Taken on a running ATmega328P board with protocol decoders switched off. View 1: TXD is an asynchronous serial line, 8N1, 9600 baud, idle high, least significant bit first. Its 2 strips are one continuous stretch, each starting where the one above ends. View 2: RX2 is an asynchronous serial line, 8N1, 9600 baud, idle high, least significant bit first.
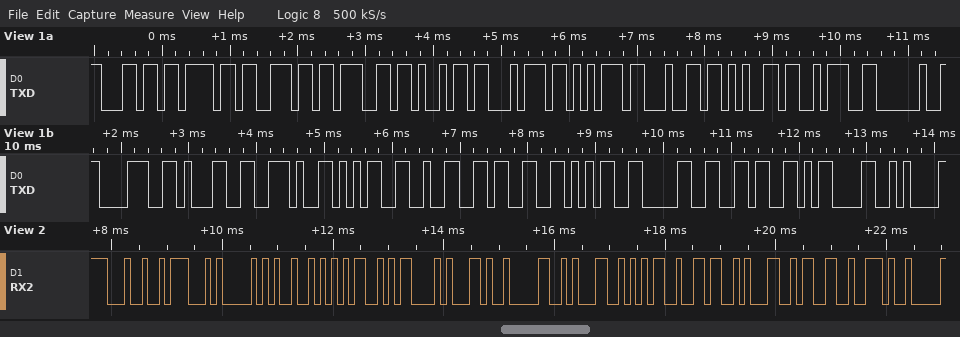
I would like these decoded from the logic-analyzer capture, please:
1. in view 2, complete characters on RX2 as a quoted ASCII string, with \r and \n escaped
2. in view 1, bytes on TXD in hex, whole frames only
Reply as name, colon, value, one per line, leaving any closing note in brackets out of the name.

in view 2, complete characters on RX2 as a quoted ASCII string, with \r and \n escaped: "$GPRMC,015613."
in view 1, bytes on TXD in hex, whole frames only: 6C 6F 6E 67 69 74 75 64 65 3A 20 38 31 2E 35 32 33 35 30 36 0D 0A
